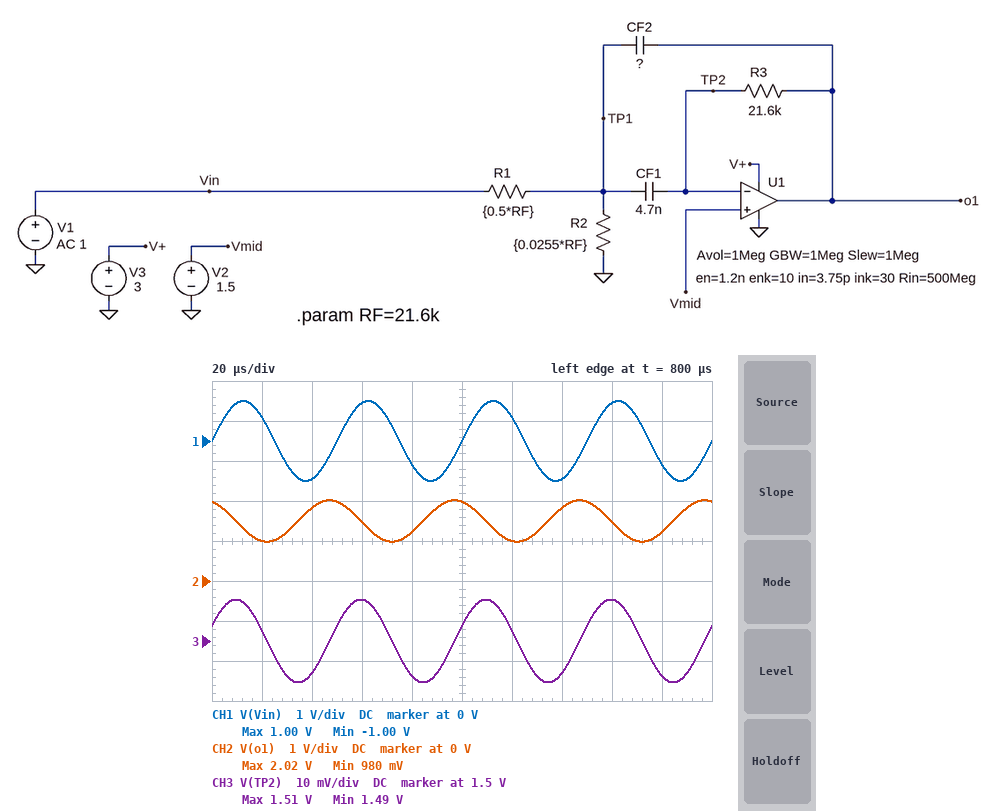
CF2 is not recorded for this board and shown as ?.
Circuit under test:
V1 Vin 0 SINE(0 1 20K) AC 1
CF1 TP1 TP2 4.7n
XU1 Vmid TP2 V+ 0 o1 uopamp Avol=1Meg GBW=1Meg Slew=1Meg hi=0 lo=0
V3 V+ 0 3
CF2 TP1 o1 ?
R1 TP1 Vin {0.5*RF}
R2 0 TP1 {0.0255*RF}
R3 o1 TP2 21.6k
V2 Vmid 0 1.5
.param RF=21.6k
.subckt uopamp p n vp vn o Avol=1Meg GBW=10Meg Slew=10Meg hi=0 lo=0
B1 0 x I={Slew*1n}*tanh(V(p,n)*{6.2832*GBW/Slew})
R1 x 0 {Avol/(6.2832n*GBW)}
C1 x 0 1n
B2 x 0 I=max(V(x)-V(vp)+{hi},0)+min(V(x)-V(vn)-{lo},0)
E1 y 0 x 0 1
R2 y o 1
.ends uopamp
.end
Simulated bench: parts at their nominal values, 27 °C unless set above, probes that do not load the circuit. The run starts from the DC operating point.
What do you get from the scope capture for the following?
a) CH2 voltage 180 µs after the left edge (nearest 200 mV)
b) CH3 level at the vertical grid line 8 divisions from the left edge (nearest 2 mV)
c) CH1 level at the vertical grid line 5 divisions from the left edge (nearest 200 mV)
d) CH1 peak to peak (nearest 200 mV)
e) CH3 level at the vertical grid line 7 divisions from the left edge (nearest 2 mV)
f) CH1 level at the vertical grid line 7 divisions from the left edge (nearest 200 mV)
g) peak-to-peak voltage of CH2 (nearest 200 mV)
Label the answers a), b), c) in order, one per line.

a) 1.2 V
b) 1.510 V
c) 0 V
d) 2.0 V
e) 1.492 V
f) -1.0 V
g) 1.0 V
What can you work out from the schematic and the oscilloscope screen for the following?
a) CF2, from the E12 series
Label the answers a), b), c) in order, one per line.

a) 2.2 nF
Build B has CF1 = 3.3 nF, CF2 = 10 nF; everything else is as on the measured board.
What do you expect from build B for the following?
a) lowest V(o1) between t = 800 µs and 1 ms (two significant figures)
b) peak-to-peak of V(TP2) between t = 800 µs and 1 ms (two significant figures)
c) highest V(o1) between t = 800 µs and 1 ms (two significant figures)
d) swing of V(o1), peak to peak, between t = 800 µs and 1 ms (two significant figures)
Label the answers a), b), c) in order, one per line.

a) 1.4 V
b) 3.4 mV
c) 1.6 V
d) 170 mV
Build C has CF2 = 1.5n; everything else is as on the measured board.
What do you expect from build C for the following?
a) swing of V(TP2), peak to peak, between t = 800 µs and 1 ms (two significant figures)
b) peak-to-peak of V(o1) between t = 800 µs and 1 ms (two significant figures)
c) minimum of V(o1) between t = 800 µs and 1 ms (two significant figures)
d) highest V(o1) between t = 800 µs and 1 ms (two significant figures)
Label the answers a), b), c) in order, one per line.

a) 38 mV
b) 1.9 V
c) 560 mV
d) 2.4 V
